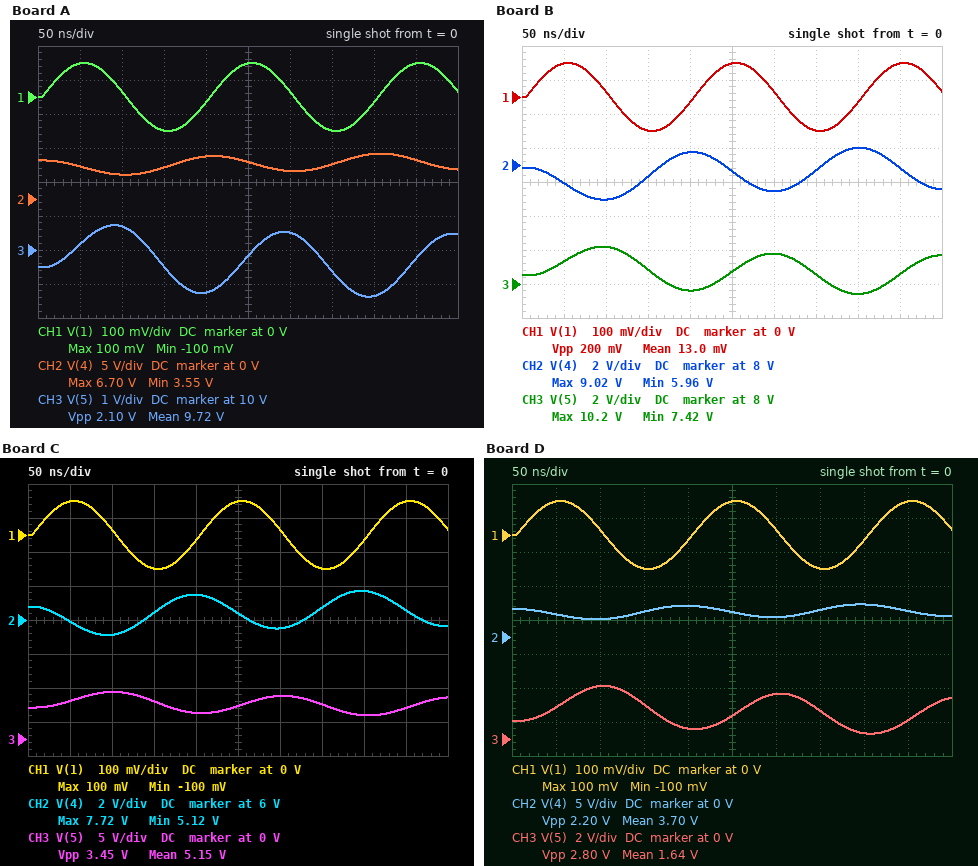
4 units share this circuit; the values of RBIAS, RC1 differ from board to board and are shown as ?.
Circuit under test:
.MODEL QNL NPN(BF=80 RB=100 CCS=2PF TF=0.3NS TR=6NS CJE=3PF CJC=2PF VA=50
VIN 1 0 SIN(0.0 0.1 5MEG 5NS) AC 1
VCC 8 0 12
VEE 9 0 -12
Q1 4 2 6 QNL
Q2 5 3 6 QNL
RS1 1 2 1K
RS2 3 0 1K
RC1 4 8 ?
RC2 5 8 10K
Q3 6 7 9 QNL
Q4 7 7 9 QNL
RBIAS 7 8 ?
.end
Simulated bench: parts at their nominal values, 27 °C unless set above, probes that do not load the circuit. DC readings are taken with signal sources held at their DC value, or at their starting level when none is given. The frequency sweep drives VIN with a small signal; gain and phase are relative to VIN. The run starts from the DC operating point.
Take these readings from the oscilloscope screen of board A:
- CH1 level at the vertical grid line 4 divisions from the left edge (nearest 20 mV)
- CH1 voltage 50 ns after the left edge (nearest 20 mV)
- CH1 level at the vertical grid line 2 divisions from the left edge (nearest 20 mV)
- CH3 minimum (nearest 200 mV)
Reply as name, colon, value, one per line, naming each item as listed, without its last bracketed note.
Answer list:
CH1 level at the vertical grid line 4 divisions from the left edge: -20 mV
CH1 voltage 50 ns after the left edge: 100 mV
CH1 level at the vertical grid line 2 divisions from the left edge: 20 mV
CH3 minimum: 8.6 V
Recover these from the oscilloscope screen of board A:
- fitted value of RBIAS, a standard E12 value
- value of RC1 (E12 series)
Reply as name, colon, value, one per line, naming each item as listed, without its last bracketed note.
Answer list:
fitted value of RBIAS, a standard E12 value: 56 kΩ
value of RC1: 27 kΩ
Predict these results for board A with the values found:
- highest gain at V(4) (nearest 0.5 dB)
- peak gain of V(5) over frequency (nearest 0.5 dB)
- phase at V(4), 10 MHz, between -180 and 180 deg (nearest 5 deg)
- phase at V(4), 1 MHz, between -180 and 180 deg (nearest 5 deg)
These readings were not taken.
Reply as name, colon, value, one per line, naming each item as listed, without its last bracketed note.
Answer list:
highest gain at V(4): 40.5 dB
peak gain of V(5) over frequency: 32.0 dB
phase at V(4), 10 MHz, between -180 and 180 deg: 80 deg
phase at V(4), 1 MHz, between -180 and 180 deg: 120 deg
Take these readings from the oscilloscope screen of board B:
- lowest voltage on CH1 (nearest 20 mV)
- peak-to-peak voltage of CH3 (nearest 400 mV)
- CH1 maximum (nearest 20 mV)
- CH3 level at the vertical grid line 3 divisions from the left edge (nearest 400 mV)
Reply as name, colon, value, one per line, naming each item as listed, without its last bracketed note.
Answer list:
lowest voltage on CH1: -100 mV
peak-to-peak voltage of CH3: 2.8 V
CH1 maximum: 100 mV
CH3 level at the vertical grid line 3 divisions from the left edge: 8.8 V
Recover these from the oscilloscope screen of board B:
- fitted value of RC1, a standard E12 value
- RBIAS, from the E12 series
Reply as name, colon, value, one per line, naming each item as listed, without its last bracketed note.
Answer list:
fitted value of RC1, a standard E12 value: 12 kΩ
RBIAS, from the E12 series: 39 kΩ
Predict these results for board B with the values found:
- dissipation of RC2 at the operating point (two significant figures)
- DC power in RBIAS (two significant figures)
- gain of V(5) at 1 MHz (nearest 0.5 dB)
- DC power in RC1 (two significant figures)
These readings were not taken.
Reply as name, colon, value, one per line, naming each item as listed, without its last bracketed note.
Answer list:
dissipation of RC2 at the operating point: 1.2 mW
DC power in RBIAS: 14 mW
gain of V(5) at 1 MHz: 32.0 dB
DC power in RC1: 1.4 mW
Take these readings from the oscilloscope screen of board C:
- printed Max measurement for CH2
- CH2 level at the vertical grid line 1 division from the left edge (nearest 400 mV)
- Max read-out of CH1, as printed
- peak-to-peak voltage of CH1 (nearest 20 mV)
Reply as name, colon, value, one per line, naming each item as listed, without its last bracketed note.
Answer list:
printed Max measurement for CH2: 7.72 V
CH2 level at the vertical grid line 1 division from the left edge: 6.0 V
Max read-out of CH1, as printed: 100 mV
peak-to-peak voltage of CH1: 200 mV
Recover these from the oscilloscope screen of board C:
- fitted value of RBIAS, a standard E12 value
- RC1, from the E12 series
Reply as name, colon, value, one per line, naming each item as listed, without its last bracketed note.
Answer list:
fitted value of RBIAS, a standard E12 value: 18 kΩ
RC1, from the E12 series: 6.8 kΩ
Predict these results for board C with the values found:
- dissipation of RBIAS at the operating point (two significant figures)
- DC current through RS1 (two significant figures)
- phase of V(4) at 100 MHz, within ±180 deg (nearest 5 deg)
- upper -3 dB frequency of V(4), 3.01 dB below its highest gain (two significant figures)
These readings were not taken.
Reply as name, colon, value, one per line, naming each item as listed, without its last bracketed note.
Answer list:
dissipation of RBIAS at the operating point: 30 mW
DC current through RS1: 8.4 µA
phase of V(4) at 100 MHz, within ±180 deg: 55 deg
upper -3 dB frequency of V(4), 3.01 dB below its highest gain: 760 kHz
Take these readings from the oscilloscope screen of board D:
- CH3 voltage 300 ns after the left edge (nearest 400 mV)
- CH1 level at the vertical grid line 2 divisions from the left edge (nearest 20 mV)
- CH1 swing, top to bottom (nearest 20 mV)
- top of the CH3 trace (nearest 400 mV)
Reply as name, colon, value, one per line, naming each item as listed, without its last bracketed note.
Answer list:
CH3 voltage 300 ns after the left edge: 2.8 V
CH1 level at the vertical grid line 2 divisions from the left edge: 20 mV
CH1 swing, top to bottom: 200 mV
top of the CH3 trace: 3.2 V
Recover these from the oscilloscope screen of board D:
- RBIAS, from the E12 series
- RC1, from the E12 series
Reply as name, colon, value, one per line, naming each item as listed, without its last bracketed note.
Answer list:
RBIAS, from the E12 series: 12 kΩ
RC1, from the E12 series: 6.8 kΩ
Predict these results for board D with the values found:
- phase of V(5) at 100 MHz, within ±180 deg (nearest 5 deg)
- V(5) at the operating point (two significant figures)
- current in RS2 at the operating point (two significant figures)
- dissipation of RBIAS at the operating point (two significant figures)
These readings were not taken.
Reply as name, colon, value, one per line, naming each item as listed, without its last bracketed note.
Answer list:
phase of V(5) at 100 MHz, within ±180 deg: -115 deg
V(5) at the operating point: 1.1 V
current in RS2 at the operating point: 13 µA
dissipation of RBIAS at the operating point: 45 mW
